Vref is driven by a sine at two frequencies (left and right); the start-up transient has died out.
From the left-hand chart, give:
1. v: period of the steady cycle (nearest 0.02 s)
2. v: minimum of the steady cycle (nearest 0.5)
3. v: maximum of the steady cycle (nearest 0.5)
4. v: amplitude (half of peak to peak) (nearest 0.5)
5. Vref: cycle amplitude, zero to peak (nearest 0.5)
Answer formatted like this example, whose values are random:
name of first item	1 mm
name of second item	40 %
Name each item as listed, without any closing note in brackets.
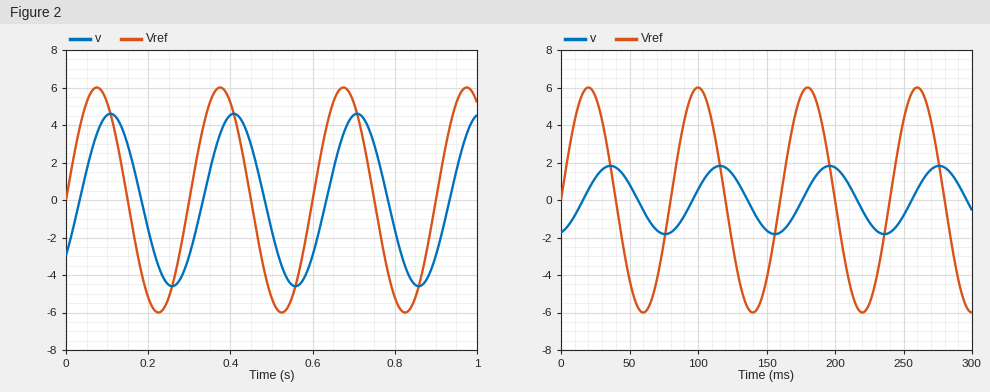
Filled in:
v: period of the steady cycle	0.30 s
v: minimum of the steady cycle	-4.5
v: maximum of the steady cycle	4.5
v: amplitude (half of peak to peak)	4.5
Vref: cycle amplitude, zero to peak	6.0
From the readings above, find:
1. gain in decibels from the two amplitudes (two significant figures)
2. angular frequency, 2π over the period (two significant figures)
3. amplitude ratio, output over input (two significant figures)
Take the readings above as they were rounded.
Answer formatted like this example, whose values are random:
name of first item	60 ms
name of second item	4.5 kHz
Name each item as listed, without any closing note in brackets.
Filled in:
gain in decibels from the two amplitudes	-2.5 dB
angular frequency, 2π over the period	21 rad/s
amplitude ratio, output over input	0.75
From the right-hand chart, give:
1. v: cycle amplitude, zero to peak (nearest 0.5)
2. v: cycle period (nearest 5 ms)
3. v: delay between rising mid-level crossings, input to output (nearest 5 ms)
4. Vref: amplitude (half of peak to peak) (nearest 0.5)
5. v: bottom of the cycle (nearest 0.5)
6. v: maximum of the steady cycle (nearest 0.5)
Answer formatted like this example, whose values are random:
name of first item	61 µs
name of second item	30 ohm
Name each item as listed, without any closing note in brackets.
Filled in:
v: cycle amplitude, zero to peak	2.0
v: cycle period	80 ms
v: delay between rising mid-level crossings, input to output	15 ms
Vref: amplitude (half of peak to peak)	6.0
v: bottom of the cycle	-2.0
v: maximum of the steady cycle	2.0
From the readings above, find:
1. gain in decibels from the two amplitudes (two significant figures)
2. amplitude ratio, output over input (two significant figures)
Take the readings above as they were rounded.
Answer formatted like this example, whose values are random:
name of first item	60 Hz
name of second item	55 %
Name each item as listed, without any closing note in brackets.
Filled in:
gain in decibels from the two amplitudes	-9.5 dB
amplitude ratio, output over input	0.33
